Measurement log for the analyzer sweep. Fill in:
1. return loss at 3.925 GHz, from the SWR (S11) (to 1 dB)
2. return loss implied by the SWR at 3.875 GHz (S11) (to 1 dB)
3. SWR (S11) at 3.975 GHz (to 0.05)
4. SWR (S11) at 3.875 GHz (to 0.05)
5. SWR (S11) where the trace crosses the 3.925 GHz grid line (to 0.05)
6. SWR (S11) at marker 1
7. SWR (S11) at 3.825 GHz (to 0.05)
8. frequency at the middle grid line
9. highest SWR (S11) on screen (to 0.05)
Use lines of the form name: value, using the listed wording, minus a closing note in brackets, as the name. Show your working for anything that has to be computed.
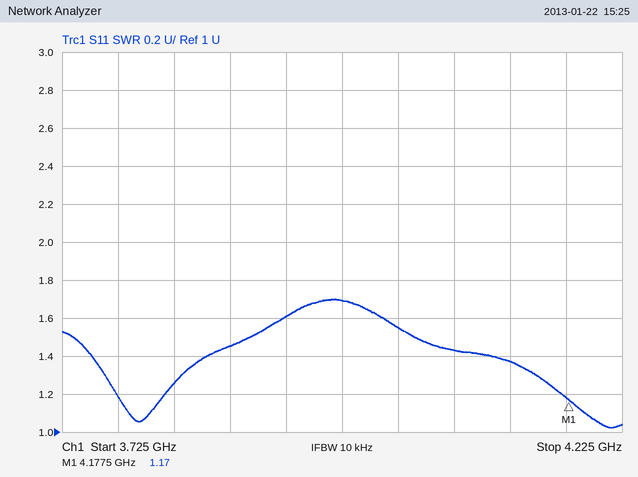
return loss at 3.925 GHz, from the SWR (S11): −20 log10((1.6 − 1)/(1.6 + 1)) ≈ 13 dB
return loss implied by the SWR at 3.875 GHz (S11): −20 log10((1.45 − 1)/(1.45 + 1)) ≈ 15 dB
SWR (S11) at 3.975 GHz: 1.70
SWR (S11) at 3.875 GHz: 1.45
SWR (S11) where the trace crosses the 3.925 GHz grid line: 1.60
SWR (S11) at marker 1: 1.17
SWR (S11) at 3.825 GHz: 1.25
frequency at the middle grid line: 3.975 GHz
highest SWR (S11) on screen: 1.70
